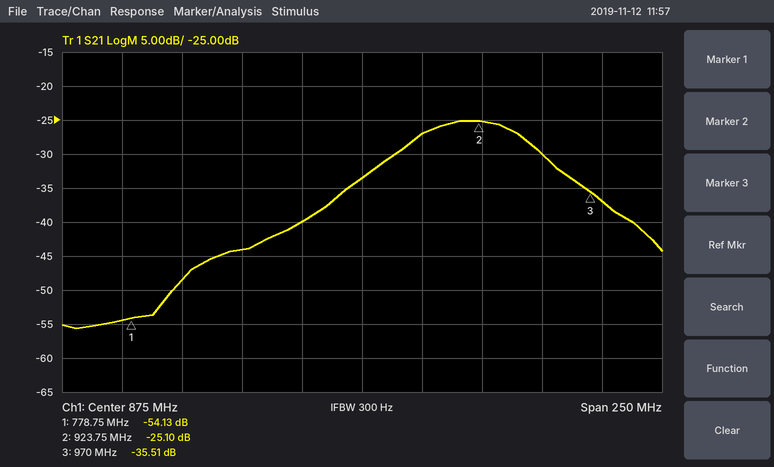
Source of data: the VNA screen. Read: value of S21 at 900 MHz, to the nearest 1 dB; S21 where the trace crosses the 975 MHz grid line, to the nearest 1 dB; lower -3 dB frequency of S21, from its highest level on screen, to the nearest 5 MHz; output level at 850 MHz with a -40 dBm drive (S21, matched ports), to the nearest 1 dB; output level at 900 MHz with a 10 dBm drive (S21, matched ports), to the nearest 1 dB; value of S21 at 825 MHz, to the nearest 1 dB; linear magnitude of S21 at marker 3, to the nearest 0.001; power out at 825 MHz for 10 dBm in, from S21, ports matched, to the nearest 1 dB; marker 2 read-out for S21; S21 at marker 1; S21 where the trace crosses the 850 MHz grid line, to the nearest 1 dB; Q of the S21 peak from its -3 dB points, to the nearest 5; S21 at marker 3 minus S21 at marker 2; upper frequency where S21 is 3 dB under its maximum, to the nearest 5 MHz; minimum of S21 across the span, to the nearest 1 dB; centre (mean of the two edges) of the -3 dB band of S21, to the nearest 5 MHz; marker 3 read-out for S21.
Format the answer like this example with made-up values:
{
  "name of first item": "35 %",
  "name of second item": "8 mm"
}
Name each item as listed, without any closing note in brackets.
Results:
{
  "value of S21 at 900 MHz, to the nearest 1 dB": "-27 dB",
  "S21 where the trace crosses the 975 MHz grid line, to the nearest 1 dB": "-37 dB",
  "lower -3 dB frequency of S21, from its highest level on screen, to the nearest 5 MHz": "895 MHz",
  "output level at 850 MHz with a -40 dBm drive (S21, matched ports), to the nearest 1 dB": "-80 dBm",
  "output level at 900 MHz with a 10 dBm drive (S21, matched ports), to the nearest 1 dB": "-17 dBm",
  "value of S21 at 825 MHz, to the nearest 1 dB": "-44 dB",
  "linear magnitude of S21 at marker 3, to the nearest 0.001": "0.017",
  "power out at 825 MHz for 10 dBm in, from S21, ports matched, to the nearest 1 dB": "-34 dBm",
  "marker 2 read-out for S21": "-25.10 dB",
  "S21 at marker 1": "-54.13 dB",
  "S21 where the trace crosses the 850 MHz grid line, to the nearest 1 dB": "-40 dB",
  "Q of the S21 peak from its -3 dB points, to the nearest 5": "20",
  "S21 at marker 3 minus S21 at marker 2": "-10.41 dB",
  "upper frequency where S21 is 3 dB under its maximum, to the nearest 5 MHz": "945 MHz",
  "minimum of S21 across the span, to the nearest 1 dB": "-56 dB",
  "centre (mean of the two edges) of the -3 dB band of S21, to the nearest 5 MHz": "920 MHz",
  "marker 3 read-out for S21": "-35.51 dB"
}
